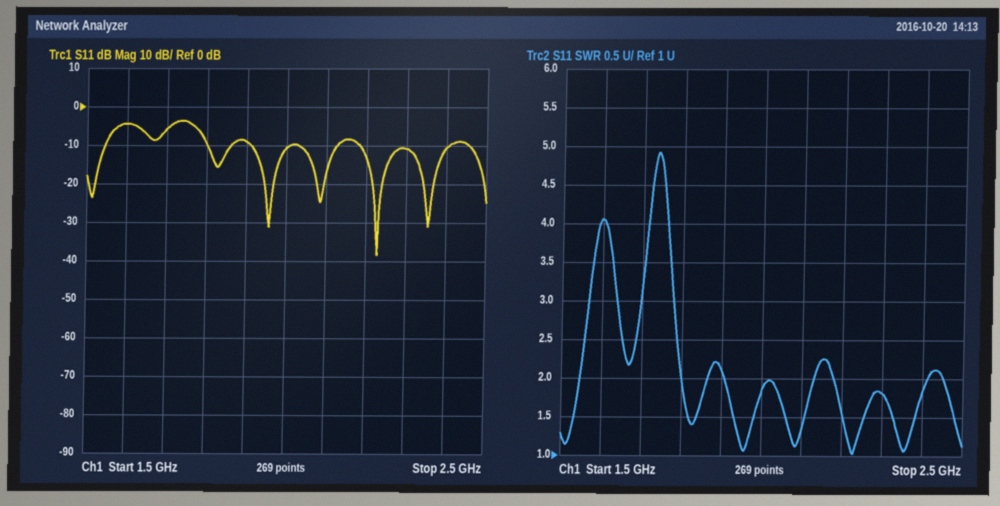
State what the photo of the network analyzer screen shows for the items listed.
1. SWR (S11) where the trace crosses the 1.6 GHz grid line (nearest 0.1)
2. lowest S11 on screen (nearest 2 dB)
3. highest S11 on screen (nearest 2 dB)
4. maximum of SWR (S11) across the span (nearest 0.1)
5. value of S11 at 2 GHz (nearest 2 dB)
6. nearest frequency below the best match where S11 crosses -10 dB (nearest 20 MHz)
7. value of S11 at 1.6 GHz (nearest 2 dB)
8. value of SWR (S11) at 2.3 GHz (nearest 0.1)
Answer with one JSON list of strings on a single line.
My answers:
["4.1", "-38 dB", "-4 dB", "4.9", "-10 dB", "2.18 GHz", "-4 dB", "1.8"]
